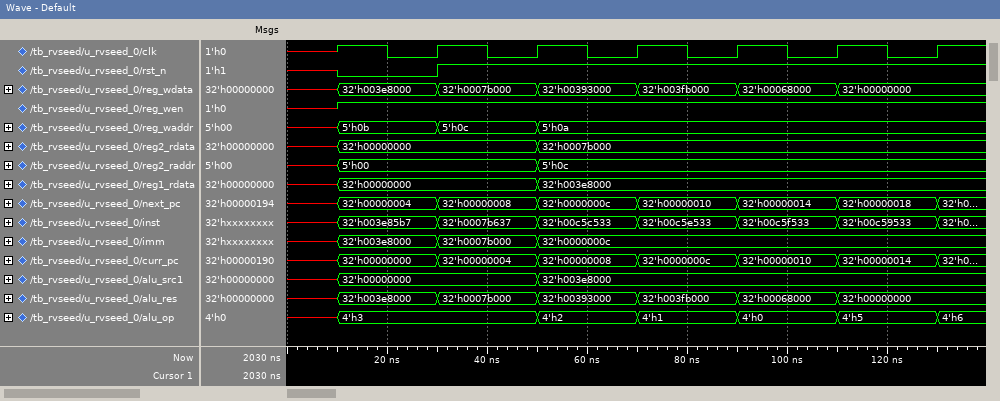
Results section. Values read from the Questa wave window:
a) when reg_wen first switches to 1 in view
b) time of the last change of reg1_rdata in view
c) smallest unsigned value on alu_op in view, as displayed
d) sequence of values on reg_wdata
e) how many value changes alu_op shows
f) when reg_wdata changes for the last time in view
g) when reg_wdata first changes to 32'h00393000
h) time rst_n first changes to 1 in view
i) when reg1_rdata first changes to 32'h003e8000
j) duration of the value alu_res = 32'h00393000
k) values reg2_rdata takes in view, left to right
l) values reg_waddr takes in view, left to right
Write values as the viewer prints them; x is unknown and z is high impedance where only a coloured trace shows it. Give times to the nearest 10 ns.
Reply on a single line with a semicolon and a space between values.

10 ns; 50 ns; 4'h0; x, 32'h003e8000, 32'h0007b000, 32'h00393000, 32'h003fb000, 32'h00068000, 32'h00000000; 6; 110 ns; 50 ns; 30 ns; 50 ns; 20 ns; x, 32'h00000000, 32'h0007b000; x, 5'h0b, 5'h0c, 5'h0a
